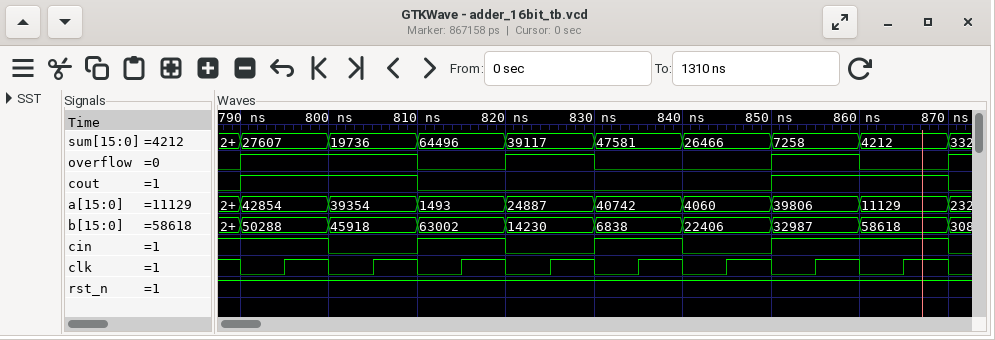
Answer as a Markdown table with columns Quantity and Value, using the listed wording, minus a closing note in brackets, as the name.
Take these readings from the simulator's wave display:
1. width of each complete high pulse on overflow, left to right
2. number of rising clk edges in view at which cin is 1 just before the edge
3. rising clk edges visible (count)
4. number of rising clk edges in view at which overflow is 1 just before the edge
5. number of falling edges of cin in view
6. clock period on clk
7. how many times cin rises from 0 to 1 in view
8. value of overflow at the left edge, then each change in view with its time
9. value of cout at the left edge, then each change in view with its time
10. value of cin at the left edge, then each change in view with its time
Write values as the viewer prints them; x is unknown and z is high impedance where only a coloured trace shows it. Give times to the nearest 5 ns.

| Quantity | Value |
|---|---|
| width of each complete high pulse on overflow, left to right | 20 ns, 10 ns, 10 ns |
| number of rising clk edges in view at which cin is 1 just before the edge | 5 |
| rising clk edges visible | 8 |
| number of rising clk edges in view at which overflow is 1 just before the edge | 4 |
| number of falling edges of cin in view | 4 |
| clock period on clk | 10 ns |
| how many times cin rises from 0 to 1 in view | 3 |
| value of overflow at the left edge, then each change in view with its time | 0, 1 at 790 ns, 0 at 810 ns, 1 at 820 ns, 0 at 830 ns, 1 at 850 ns, 0 at 860 ns, 1 at 870 ns |
| value of cout at the left edge, then each change in view with its time | 0, 1 at 790 ns, 0 at 810 ns, 1 at 850 ns, 0 at 870 ns |
| value of cin at the left edge, then each change in view with its time | 1, 0 at 800 ns, 1 at 810 ns, 0 at 820 ns, 1 at 830 ns, 0 at 840 ns, 1 at 850 ns, 0 at 870 ns |
